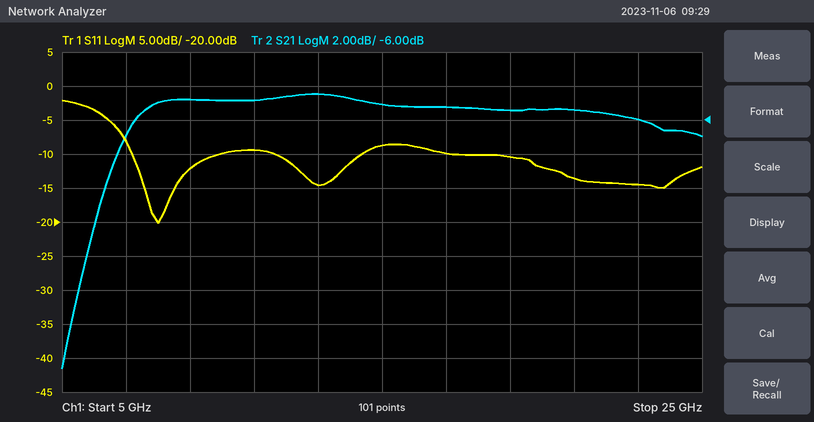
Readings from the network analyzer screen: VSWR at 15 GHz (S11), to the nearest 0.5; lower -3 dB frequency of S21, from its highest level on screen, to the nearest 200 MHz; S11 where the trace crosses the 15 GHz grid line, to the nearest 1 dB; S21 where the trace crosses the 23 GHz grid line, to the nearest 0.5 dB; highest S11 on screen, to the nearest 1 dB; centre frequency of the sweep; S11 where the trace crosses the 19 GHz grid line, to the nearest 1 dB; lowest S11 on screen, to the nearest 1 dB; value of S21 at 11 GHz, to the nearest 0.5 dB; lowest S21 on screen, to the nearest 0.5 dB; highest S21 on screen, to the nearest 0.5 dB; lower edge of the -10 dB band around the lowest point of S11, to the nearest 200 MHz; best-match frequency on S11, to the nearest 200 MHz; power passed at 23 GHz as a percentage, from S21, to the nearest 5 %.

2.0
6.8 GHz
-9 dB
-6.0 dB
-2 dB
15 GHz
-10 dB
-20 dB
-5.0 dB
-20.5 dB
-4.5 dB
7.2 GHz
8.0 GHz
25 %
